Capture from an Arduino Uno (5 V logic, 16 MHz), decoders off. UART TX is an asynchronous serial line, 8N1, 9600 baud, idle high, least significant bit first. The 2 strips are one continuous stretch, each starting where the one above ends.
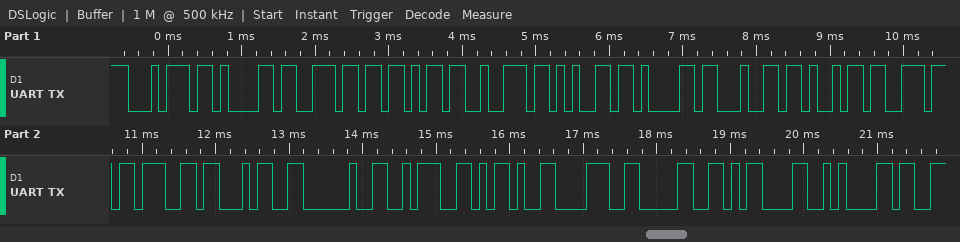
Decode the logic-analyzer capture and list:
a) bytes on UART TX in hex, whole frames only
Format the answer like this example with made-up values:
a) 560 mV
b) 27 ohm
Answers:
a) 0x74 0x61 0x6E 0x6B 0x72 0x65 0x61 0x64 0x69 0x6E 0x67 0x34 0x20 0x3A 0x2D 0x38 0x30 0x0D 0x0A
